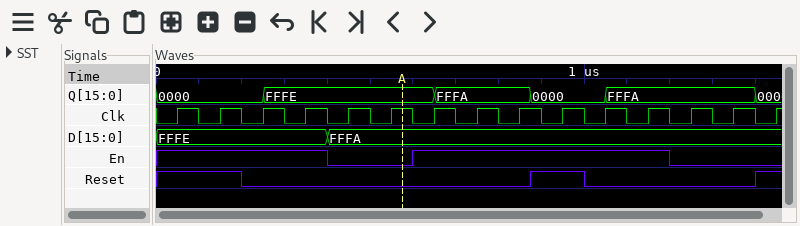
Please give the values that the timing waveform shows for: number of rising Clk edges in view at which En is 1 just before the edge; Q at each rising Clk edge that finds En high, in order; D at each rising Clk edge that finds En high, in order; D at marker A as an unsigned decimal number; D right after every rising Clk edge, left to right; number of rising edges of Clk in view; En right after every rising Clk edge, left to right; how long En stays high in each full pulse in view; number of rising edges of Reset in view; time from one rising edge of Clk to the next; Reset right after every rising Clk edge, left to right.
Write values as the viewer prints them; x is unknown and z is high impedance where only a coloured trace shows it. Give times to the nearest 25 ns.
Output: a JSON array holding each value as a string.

["10", "0000, 0000, 0000, FFFE, FFFE, FFFA, FFFA, 0000, 0000, FFFA", "FFFE, FFFE, FFFE, FFFE, FFFA, FFFA, FFFA, FFFA, FFFA, FFFA", "65530", "FFFE, FFFE, FFFE, FFFE, FFFA, FFFA, FFFA, FFFA, FFFA, FFFA, FFFA, FFFA, FFFA, FFFA, FFFA", "15", "1 1 1 1 0 0 1 1 1 1 1 1 0 0 0", "600 ns", "2", "100 ns", "1 1 0 0 0 0 0 0 0 1 0 0 0 0 1"]
